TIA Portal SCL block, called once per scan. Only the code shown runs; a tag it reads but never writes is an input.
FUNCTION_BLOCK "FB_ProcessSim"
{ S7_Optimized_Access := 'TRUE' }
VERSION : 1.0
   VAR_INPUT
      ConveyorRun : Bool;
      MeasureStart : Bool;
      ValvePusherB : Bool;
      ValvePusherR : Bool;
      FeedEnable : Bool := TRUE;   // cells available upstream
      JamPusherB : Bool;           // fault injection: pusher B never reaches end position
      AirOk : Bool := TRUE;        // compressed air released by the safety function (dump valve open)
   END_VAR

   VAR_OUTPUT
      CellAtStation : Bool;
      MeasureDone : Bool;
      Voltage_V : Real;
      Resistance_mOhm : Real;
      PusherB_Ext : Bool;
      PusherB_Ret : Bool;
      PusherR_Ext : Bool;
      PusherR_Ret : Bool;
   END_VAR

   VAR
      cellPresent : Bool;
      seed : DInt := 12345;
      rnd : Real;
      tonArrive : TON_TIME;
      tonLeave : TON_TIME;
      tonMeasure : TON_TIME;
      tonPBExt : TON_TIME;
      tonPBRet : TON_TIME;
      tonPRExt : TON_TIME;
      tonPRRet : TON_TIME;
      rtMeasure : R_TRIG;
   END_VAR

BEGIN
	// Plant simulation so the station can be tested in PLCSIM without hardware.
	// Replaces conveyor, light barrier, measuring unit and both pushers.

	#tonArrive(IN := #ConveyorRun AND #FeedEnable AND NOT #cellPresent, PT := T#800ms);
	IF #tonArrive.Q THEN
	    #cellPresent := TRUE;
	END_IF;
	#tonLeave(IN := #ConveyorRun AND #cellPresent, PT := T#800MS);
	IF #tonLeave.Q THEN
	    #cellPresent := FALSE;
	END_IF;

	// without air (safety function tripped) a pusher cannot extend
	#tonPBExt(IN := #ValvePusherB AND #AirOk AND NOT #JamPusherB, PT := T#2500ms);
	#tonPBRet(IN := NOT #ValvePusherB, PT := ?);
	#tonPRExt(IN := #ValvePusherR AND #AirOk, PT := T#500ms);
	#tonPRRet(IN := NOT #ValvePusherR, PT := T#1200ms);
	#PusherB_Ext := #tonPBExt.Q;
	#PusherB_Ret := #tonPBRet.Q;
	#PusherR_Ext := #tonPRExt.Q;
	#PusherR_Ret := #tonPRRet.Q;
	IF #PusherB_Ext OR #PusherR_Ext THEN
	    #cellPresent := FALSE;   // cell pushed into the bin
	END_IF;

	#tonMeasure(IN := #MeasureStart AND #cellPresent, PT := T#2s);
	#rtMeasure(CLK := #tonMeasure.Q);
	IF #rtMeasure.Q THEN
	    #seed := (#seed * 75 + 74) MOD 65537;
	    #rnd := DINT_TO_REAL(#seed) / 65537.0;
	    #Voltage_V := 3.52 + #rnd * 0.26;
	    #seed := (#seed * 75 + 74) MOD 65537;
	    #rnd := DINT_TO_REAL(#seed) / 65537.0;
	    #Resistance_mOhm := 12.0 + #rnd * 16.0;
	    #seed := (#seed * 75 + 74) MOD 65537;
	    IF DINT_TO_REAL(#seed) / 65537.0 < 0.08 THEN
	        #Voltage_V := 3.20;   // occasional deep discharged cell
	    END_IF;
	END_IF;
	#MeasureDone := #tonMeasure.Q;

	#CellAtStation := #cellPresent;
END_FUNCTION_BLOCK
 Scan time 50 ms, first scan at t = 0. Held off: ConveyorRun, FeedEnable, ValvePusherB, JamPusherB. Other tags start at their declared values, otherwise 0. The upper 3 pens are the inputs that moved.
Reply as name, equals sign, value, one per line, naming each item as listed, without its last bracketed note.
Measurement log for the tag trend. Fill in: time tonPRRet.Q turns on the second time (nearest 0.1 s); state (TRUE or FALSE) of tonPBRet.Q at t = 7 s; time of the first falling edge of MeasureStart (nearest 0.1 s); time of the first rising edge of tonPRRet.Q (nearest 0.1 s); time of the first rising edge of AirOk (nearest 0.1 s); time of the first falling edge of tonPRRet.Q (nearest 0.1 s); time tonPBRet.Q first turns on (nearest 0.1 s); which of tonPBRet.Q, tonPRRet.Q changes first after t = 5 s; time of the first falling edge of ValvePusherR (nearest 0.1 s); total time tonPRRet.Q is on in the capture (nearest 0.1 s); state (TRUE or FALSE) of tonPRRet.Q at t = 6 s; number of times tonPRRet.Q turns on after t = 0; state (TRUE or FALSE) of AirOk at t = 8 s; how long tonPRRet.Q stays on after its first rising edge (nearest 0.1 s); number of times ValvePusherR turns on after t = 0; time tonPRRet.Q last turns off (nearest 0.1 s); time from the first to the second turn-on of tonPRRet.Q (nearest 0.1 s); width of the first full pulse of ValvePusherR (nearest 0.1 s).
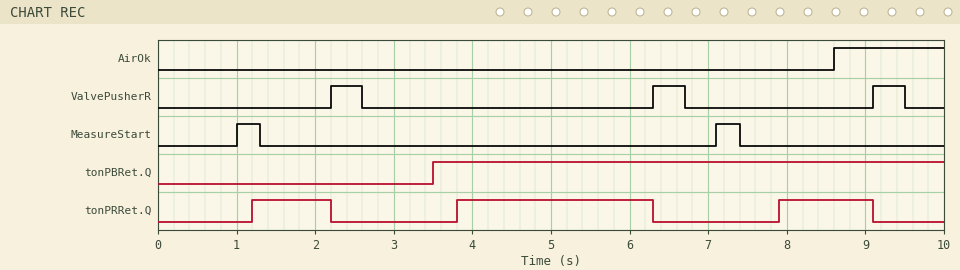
time tonPRRet.Q turns on the second time = 3.8 s
state (TRUE or FALSE) of tonPBRet.Q at t = 7 s = TRUE
time of the first falling edge of MeasureStart = 1.3 s
time of the first rising edge of tonPRRet.Q = 1.2 s
time of the first rising edge of AirOk = 8.6 s
time of the first falling edge of tonPRRet.Q = 2.2 s
time tonPBRet.Q first turns on = 3.5 s
which of tonPBRet.Q, tonPRRet.Q changes first after t = 5 s = tonPRRet.Q
time of the first falling edge of ValvePusherR = 2.6 s
total time tonPRRet.Q is on in the capture = 4.7 s
state (TRUE or FALSE) of tonPRRet.Q at t = 6 s = TRUE
number of times tonPRRet.Q turns on after t = 0 = 3
state (TRUE or FALSE) of AirOk at t = 8 s = FALSE
how long tonPRRet.Q stays on after its first rising edge = 1.0 s
number of times ValvePusherR turns on after t = 0 = 3
time tonPRRet.Q last turns off = 9.1 s
time from the first to the second turn-on of tonPRRet.Q = 2.6 s
width of the first full pulse of ValvePusherR = 0.4 s
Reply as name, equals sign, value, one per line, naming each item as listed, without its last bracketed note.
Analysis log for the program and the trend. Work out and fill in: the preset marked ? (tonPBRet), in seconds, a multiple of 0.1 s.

the preset marked ? (tonPBRet), in seconds, a multiple of 0.1 s = 3.5 s
